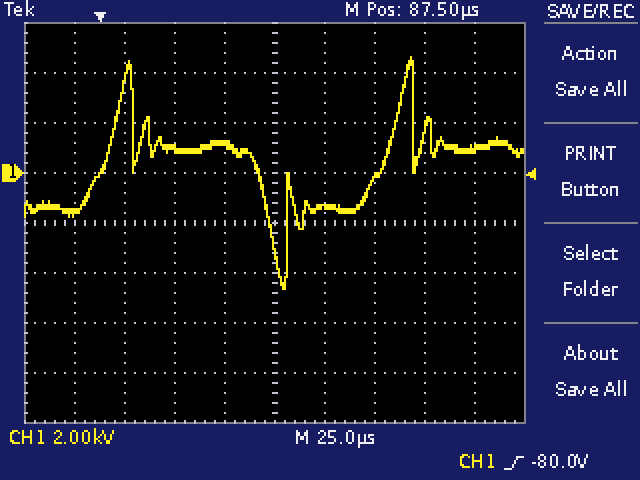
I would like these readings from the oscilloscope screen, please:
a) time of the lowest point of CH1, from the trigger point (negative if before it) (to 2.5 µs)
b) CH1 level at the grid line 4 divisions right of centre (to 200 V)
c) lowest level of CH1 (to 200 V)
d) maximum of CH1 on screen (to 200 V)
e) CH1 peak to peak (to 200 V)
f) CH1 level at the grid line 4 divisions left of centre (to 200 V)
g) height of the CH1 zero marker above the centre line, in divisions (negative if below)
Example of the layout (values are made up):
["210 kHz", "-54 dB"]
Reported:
["+92.5 µs", "1.0 kV", "-4.6 kV", "4.6 kV", "9.2 kV", "-1.6 kV", "+1.0 div"]
